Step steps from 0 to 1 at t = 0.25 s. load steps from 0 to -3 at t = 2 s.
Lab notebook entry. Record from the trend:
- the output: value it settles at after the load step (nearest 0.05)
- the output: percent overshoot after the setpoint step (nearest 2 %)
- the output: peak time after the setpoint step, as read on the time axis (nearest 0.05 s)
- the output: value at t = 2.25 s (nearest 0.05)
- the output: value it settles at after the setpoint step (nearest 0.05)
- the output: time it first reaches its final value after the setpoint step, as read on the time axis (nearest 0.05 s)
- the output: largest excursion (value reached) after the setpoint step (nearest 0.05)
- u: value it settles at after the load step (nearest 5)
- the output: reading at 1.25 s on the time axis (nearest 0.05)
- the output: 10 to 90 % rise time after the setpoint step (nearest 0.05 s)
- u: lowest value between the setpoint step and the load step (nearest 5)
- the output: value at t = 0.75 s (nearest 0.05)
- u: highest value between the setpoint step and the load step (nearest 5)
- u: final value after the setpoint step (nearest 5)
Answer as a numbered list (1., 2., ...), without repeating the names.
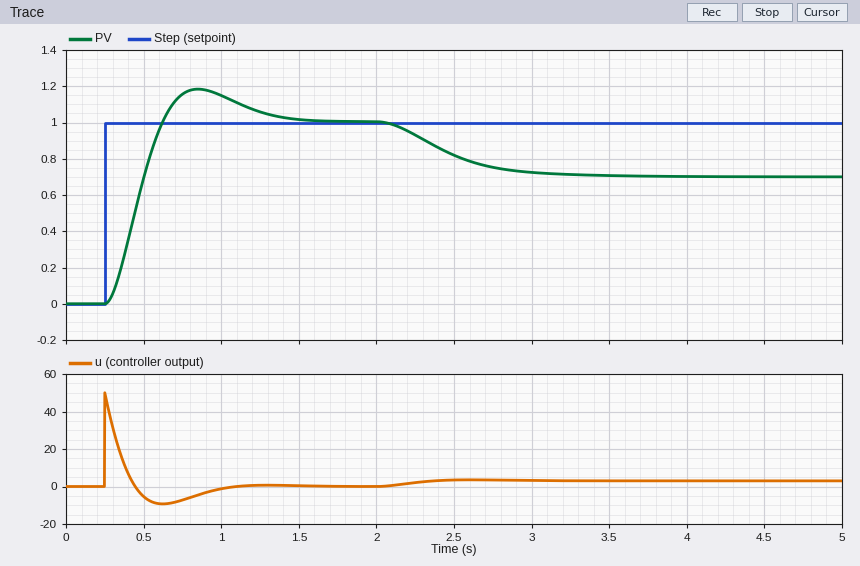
1. 0.70
2. 18 %
3. 0.85 s
4. 0.95
5. 1.00
6. 0.60 s
7. 1.20
8. 5
9. 1.05
10. 0.25 s
11. -10
12. 1.15
13. 50
14. 0
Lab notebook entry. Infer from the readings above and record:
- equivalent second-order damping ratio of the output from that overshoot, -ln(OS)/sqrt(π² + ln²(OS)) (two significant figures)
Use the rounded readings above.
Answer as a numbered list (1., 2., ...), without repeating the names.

1. 0.48
